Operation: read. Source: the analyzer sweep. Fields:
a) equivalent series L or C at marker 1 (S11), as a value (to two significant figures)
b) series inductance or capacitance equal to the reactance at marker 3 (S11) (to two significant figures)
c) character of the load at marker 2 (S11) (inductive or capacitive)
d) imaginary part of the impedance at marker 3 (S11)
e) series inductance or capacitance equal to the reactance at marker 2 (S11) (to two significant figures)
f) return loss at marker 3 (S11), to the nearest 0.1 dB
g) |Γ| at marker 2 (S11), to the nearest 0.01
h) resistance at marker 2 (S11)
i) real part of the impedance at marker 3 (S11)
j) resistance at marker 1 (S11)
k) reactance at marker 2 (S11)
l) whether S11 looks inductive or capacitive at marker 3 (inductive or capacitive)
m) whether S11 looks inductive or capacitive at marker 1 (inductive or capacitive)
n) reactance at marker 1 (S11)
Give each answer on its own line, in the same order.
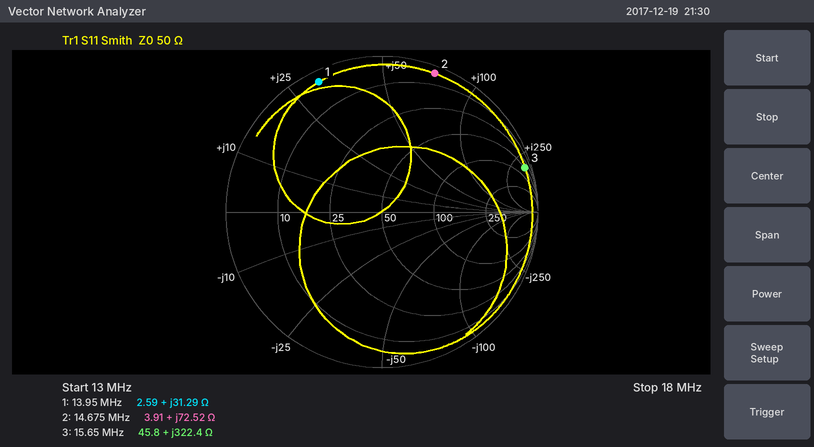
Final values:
360 nH
3.3 µH
inductive
+322.4 Ω
790 nH
0.4 dB
0.95
3.91 Ω
45.8 Ω
2.59 Ω
+72.52 Ω
inductive
inductive
+31.29 Ω
